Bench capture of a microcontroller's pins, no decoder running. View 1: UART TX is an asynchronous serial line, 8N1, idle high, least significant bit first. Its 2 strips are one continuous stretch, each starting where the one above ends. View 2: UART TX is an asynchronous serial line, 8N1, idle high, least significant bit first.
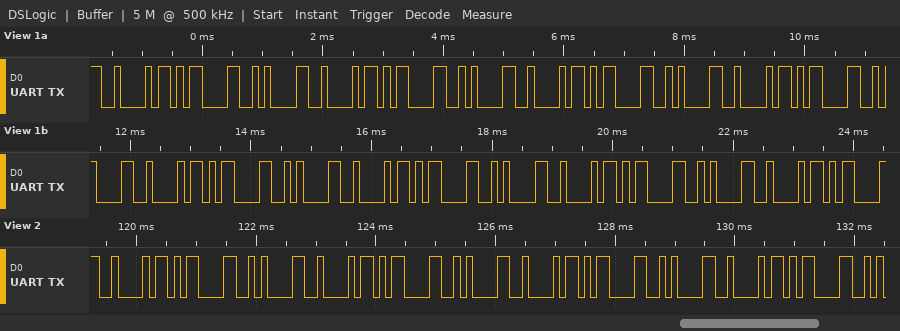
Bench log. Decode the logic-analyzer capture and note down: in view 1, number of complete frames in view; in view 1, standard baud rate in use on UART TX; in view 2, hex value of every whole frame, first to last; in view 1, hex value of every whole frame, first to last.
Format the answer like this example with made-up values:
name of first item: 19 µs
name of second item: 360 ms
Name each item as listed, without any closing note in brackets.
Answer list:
in view 1, number of complete frames in view: 23
in view 1, standard baud rate in use on UART TX: 9600 baud
in view 2, hex value of every whole frame, first to last: 42 0D 0A 42 0D 0A 42 0D 0A 42 0D
in view 1, hex value of every whole frame, first to last: 42 0D 0A 42 0D 0A 42 0D 0A 42 0D 0A 42 0D 0A 42 0D 0A 42 0D 0A 42 0D
